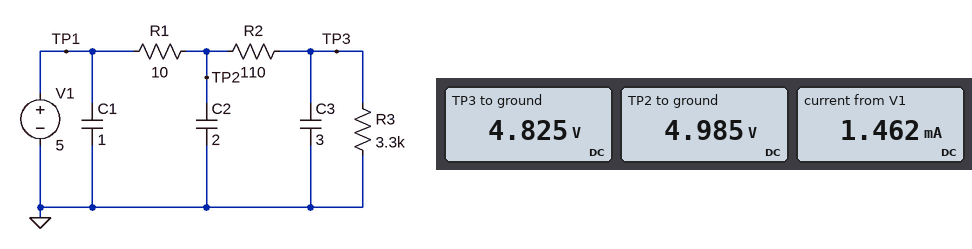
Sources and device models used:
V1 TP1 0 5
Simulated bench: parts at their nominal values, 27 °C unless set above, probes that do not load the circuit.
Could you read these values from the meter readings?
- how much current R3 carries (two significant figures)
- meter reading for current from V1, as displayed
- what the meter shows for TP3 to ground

1.5 mA
1.462 mA
4.825 V
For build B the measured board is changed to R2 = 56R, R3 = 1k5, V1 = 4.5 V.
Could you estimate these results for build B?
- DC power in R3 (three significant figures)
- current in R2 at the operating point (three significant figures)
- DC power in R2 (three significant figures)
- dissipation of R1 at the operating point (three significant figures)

12.4 mW
2.87 mA
462 µW
82.6 µW
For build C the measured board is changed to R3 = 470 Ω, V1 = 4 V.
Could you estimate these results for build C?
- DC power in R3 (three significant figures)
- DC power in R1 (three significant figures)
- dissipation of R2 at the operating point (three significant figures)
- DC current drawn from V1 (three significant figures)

21.6 mW
460 µW
5.06 mW
6.78 mA
